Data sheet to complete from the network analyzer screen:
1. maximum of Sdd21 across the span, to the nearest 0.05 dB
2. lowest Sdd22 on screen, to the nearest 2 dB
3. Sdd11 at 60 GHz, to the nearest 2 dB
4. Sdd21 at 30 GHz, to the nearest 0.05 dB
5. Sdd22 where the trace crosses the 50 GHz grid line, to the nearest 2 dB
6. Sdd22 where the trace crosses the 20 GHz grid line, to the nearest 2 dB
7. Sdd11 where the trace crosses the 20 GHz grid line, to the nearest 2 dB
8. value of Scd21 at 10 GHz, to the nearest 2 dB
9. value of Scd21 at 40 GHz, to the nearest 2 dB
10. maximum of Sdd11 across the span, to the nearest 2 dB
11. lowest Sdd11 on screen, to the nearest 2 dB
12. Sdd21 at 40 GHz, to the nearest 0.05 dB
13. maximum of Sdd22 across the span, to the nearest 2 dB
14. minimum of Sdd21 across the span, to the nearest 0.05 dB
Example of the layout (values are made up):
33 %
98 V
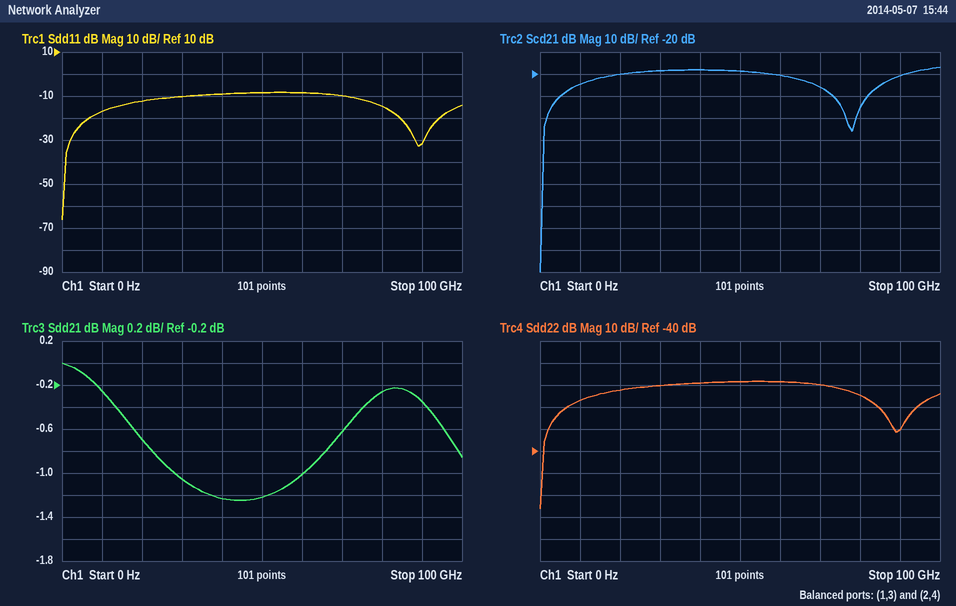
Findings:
0.00 dB
-66 dB
-8 dB
-1.05 dB
-8 dB
-12 dB
-12 dB
-24 dB
-18 dB
-8 dB
-66 dB
-1.25 dB
-8 dB
-1.25 dB
